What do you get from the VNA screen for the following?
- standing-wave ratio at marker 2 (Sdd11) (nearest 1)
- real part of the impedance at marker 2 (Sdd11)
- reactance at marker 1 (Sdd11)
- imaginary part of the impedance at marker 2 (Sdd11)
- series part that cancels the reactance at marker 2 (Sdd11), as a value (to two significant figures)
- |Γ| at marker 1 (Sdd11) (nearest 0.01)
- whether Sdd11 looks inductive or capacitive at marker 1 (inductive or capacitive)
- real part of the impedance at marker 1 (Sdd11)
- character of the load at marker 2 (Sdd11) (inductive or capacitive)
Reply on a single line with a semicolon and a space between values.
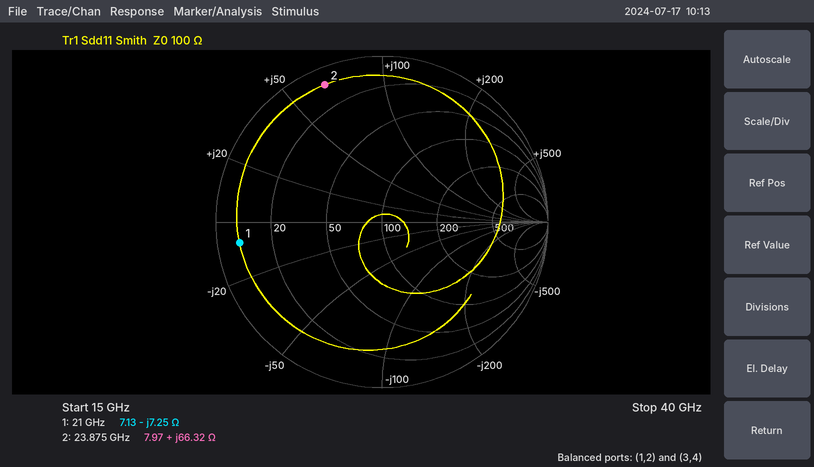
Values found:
18; 7.97 Ω; -7.25 Ω; +66.32 Ω; 100 fF; 0.87; capacitive; 7.13 Ω; inductive
